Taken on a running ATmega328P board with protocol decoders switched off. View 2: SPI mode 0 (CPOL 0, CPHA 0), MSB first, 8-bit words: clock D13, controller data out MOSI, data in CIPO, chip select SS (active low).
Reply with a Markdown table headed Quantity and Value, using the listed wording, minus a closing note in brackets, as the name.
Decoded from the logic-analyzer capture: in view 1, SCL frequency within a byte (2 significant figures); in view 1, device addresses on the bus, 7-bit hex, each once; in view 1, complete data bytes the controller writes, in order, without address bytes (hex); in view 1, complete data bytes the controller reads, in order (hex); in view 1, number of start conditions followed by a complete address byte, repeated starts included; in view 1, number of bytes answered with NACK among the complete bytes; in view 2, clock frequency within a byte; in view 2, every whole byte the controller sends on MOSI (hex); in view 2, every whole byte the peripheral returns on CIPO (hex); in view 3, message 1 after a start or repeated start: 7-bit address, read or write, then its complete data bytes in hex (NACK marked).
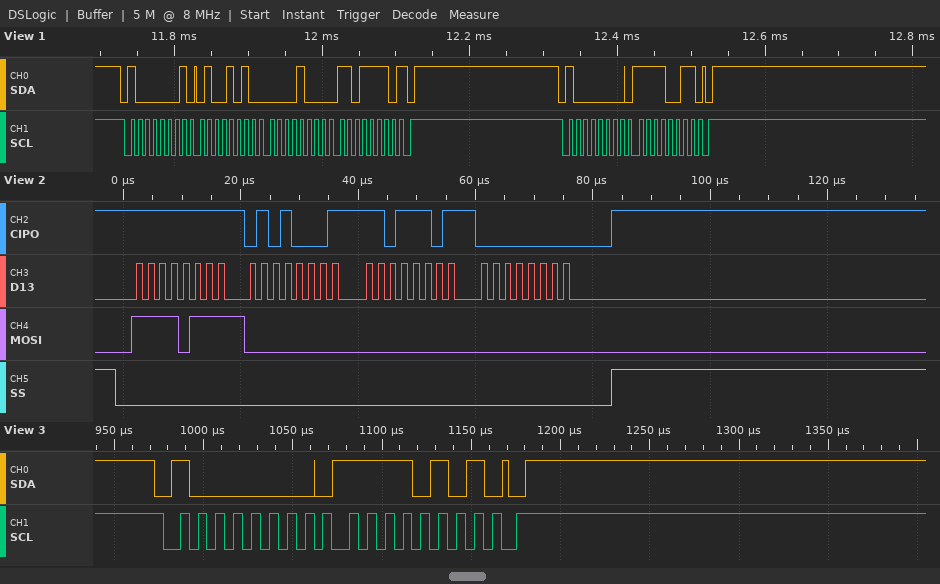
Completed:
| Quantity | Value |
|---|---|
| in view 1, SCL frequency within a byte | 100 kHz |
| in view 1, device addresses on the bus, 7-bit hex, each once | 0x40 |
| in view 1, complete data bytes the controller writes, in order, without address bytes | F3 |
| in view 1, complete data bytes the controller reads, in order | 4A 08 DE |
| in view 1, number of start conditions followed by a complete address byte, repeated starts included | 2 |
| in view 1, number of bytes answered with NACK among the complete bytes | 1 |
| in view 2, clock frequency within a byte | 500 kHz |
| in view 2, every whole byte the controller sends on MOSI | 0xF7 0x00 0x00 0x00 |
| in view 2, every whole byte the peripheral returns on CIPO | 0xFF 0x51 0xDD 0x00 |
| in view 3, message 1 after a start or repeated start: 7-bit address, read or write, then its complete data bytes in hex | 0x40 write: F5 |
